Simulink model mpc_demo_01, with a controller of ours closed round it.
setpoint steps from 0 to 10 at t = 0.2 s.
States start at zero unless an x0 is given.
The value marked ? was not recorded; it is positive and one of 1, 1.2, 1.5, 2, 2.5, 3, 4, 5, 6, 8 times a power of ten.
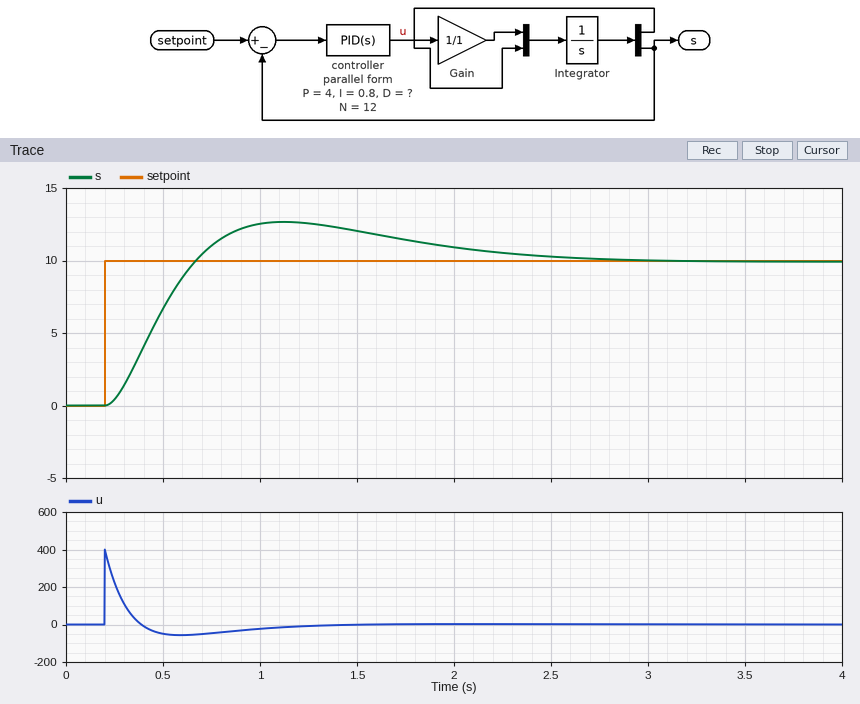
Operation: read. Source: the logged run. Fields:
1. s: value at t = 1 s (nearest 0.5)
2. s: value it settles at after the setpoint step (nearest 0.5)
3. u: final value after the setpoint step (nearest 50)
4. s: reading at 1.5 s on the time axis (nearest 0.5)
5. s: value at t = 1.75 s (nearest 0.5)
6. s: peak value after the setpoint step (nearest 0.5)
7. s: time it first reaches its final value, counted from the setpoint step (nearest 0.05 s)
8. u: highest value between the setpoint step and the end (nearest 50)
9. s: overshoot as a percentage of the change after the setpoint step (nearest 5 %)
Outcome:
12.5
10.0
0
12.0
11.5
12.5
0.45 s
400
25 %
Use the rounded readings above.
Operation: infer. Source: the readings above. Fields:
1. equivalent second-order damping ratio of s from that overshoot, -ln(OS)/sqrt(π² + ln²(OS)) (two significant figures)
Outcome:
0.40
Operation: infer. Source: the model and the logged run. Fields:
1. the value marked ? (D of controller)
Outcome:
3
